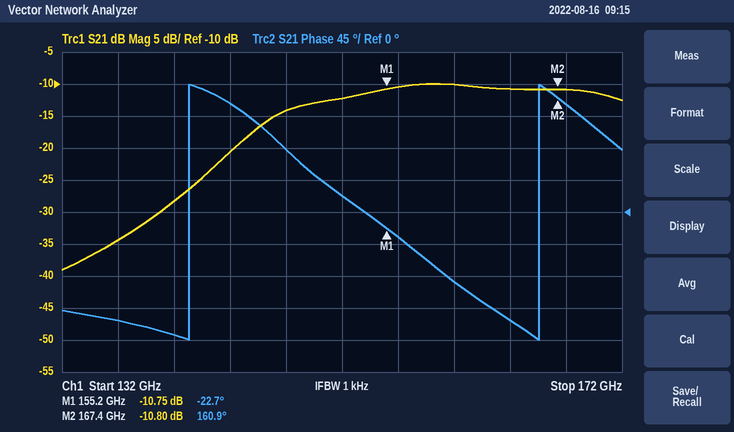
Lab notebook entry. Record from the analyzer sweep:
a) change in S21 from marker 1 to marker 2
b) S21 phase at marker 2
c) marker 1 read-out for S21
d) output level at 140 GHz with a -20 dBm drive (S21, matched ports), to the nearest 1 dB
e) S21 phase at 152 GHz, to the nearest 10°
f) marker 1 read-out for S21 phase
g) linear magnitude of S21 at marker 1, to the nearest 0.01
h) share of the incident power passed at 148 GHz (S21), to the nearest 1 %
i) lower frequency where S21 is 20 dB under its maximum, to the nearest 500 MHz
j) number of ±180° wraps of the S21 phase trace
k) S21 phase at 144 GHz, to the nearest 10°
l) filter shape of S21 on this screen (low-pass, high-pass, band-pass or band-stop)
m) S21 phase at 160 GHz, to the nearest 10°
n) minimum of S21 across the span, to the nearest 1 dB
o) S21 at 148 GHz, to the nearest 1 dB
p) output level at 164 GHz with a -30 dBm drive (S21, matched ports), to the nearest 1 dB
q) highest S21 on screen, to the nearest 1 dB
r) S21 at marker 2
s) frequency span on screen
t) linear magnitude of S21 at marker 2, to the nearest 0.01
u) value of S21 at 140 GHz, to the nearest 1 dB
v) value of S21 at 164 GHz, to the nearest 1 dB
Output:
-0.05 dB
160.9°
-10.75 dB
-48 dBm
20°
-22.7°
0.29
4 %
139.0 GHz
2
150°
high-pass
-100°
-39 dB
-14 dB
-41 dBm
-10 dB
-10.80 dB
40 GHz
0.29
-28 dB
-11 dB
